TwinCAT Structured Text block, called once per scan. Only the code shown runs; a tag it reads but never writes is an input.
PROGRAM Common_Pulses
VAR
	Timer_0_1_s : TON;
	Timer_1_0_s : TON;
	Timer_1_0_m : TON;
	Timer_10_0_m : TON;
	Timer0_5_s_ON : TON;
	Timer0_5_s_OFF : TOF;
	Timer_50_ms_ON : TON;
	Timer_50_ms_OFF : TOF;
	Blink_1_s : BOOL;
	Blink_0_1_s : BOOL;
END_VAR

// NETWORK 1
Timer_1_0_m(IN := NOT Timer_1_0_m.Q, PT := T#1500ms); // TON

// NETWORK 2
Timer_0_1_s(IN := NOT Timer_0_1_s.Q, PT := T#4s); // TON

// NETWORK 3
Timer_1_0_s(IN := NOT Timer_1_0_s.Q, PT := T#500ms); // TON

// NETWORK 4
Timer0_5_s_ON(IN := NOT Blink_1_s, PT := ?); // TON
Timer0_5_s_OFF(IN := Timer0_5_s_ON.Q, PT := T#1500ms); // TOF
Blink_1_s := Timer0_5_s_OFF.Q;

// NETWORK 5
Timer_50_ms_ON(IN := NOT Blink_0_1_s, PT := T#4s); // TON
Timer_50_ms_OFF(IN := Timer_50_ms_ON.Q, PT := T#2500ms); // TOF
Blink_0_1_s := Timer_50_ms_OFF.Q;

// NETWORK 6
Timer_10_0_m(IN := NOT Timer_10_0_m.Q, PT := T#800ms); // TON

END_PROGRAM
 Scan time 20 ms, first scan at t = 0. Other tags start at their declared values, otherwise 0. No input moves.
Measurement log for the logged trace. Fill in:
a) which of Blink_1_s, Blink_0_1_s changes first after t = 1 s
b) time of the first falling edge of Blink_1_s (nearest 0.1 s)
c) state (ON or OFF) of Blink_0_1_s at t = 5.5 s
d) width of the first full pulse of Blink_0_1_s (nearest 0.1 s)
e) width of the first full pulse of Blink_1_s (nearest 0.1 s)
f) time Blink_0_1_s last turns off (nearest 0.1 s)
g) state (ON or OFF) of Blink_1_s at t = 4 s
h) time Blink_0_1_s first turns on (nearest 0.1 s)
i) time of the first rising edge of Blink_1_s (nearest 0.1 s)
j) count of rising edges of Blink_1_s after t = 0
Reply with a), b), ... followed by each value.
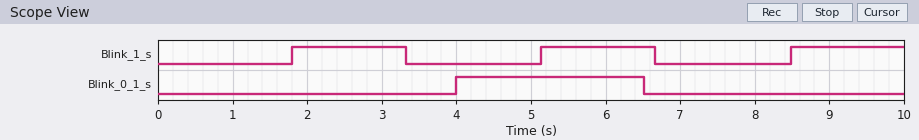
a) Blink_1_s
b) 3.3 s
c) ON
d) 2.5 s
e) 1.5 s
f) 6.5 s
g) OFF
h) 4.0 s
i) 1.8 s
j) 3
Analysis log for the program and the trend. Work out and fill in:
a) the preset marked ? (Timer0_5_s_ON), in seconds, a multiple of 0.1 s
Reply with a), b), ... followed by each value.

a) 1.8 s
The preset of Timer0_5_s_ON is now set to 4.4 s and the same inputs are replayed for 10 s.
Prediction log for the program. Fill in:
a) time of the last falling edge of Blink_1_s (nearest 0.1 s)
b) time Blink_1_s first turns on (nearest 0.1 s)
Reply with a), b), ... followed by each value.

a) 5.9 s
b) 4.4 s
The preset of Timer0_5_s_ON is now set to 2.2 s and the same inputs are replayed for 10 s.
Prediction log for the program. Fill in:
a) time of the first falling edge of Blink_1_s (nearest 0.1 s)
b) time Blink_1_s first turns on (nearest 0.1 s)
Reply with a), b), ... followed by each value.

a) 3.7 s
b) 2.2 s
